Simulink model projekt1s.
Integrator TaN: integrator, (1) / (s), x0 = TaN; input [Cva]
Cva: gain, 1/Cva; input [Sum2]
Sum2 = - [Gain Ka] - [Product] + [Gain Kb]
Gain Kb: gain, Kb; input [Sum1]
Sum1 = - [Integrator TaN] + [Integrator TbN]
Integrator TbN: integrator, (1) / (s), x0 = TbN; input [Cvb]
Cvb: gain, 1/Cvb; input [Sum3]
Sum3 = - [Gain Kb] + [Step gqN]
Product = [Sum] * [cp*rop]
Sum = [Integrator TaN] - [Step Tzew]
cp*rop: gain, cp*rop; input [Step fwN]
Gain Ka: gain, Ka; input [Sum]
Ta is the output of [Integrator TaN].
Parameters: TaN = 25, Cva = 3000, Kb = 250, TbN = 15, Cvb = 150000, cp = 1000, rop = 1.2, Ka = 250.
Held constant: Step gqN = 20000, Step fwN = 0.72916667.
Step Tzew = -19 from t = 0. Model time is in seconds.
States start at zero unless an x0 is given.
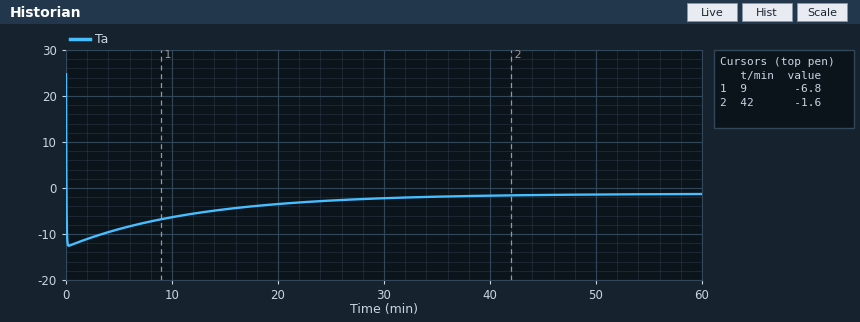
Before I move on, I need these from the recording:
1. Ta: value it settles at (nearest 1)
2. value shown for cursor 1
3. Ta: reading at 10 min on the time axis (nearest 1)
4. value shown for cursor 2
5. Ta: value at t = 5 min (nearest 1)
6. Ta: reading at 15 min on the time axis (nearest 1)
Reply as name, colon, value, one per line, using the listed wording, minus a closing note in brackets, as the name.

Ta: value it settles at: -1
value shown for cursor 1: -6.8
Ta: reading at 10 min on the time axis: -6
value shown for cursor 2: -1.6
Ta: value at t = 5 min: -9
Ta: reading at 15 min on the time axis: -5
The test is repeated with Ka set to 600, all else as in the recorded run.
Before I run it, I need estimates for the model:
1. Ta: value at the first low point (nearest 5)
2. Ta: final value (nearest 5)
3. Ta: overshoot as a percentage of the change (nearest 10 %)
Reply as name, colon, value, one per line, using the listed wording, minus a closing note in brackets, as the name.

Ta: value at the first low point: -15
Ta: final value: -5
Ta: overshoot as a percentage of the change: 30 %
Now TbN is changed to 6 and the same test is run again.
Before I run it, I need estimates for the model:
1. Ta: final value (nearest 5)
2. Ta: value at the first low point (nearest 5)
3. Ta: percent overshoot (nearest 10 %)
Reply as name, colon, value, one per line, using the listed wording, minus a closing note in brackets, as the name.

Ta: final value: 0
Ta: value at the first low point: -15
Ta: percent overshoot: 50 %
